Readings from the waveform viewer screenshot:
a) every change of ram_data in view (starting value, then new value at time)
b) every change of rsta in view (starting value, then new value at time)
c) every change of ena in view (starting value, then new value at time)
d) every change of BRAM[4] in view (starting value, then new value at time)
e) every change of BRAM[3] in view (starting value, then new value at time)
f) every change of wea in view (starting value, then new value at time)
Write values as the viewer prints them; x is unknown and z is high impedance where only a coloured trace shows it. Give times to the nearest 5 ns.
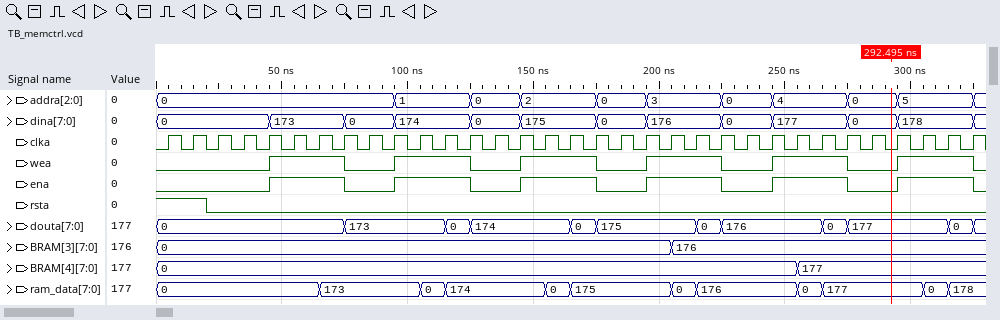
0, 173 at 65 ns, 0 at 105 ns, 174 at 115 ns, 0 at 155 ns, 175 at 165 ns, 0 at 205 ns, 176 at 215 ns, 0 at 255 ns, 177 at 265 ns, 0 at 305 ns, 178 at 315 ns
1, 0 at 20 ns
0, 1 at 45 ns, 0 at 75 ns, 1 at 95 ns, 0 at 125 ns, 1 at 145 ns, 0 at 175 ns, 1 at 195 ns, 0 at 225 ns, 1 at 245 ns, 0 at 275 ns, 1 at 295 ns, 0 at 325 ns
0, 177 at 255 ns
0, 176 at 205 ns
0, 1 at 45 ns, 0 at 75 ns, 1 at 95 ns, 0 at 125 ns, 1 at 145 ns, 0 at 175 ns, 1 at 195 ns, 0 at 225 ns, 1 at 245 ns, 0 at 275 ns, 1 at 295 ns, 0 at 325 ns
